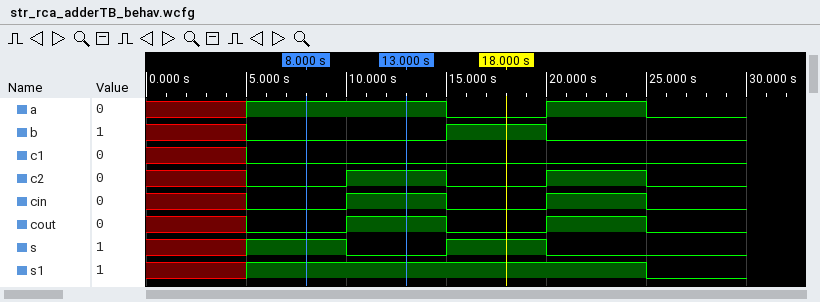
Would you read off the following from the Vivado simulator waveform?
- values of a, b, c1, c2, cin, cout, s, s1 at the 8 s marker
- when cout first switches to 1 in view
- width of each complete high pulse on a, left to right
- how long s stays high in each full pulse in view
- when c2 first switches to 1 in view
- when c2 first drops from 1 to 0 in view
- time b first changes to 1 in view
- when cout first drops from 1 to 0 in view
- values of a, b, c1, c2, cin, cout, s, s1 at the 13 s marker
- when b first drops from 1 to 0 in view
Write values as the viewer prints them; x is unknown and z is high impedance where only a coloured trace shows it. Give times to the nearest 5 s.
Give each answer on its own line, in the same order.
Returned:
a=1, b=0, c1=0, c2=0, cin=0, cout=0, s=1, s1=1
10 s
5 s
5 s
10 s
15 s
15 s
15 s
a=1, b=0, c1=0, c2=1, cin=1, cout=1, s=0, s1=1
20 s
